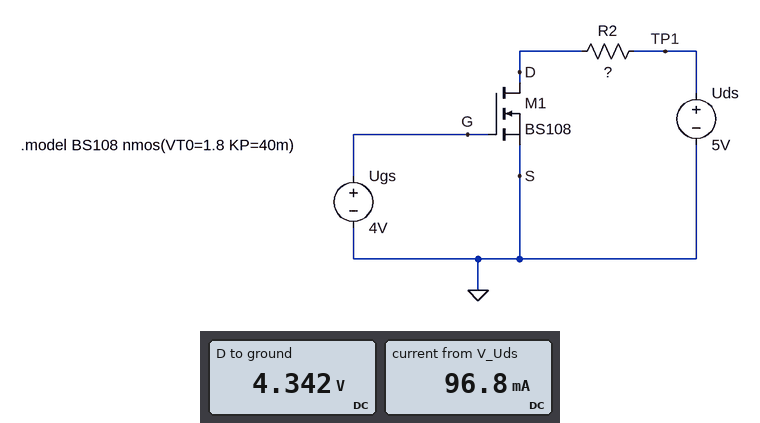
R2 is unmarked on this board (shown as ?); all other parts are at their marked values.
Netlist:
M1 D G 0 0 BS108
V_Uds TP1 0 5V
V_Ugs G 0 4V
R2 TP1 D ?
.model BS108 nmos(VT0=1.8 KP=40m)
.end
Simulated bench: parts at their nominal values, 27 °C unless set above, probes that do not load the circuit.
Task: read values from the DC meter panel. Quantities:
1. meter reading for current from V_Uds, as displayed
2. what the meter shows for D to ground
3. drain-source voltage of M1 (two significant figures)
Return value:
96.8 mA
4.342 V
4.3 V
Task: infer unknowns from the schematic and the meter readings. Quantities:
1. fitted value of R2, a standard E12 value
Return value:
6.8 Ω
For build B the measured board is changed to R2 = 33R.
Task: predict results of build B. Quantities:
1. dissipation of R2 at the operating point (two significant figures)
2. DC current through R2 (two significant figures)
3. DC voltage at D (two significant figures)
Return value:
300 mW
95 mA
1.9 V
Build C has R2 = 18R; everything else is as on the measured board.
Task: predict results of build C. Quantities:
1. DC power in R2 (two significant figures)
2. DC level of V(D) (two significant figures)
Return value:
170 mW
3.3 V
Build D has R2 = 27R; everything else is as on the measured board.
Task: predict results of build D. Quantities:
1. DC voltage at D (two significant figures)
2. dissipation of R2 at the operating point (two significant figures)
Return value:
2.4 V
250 mW
